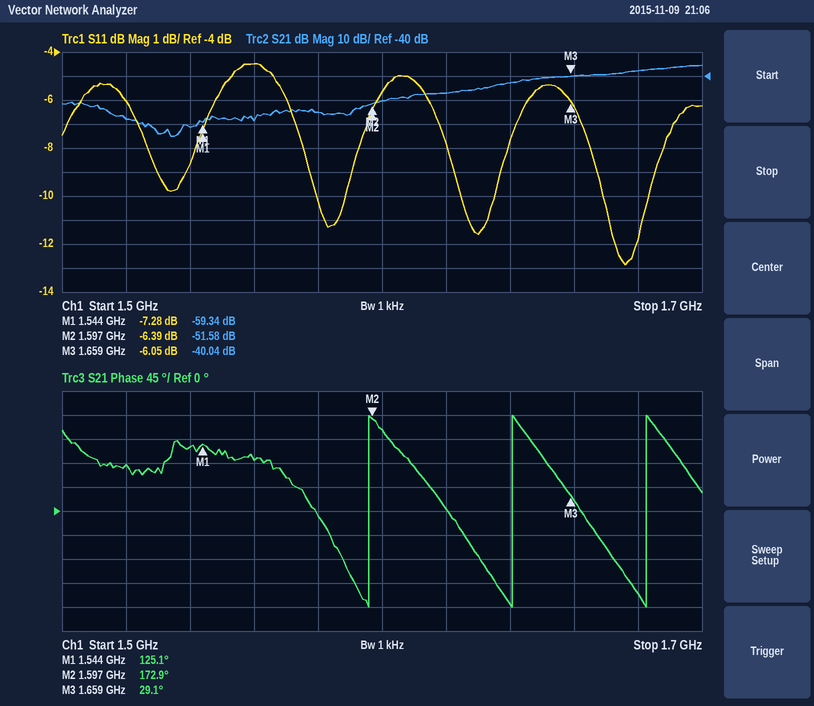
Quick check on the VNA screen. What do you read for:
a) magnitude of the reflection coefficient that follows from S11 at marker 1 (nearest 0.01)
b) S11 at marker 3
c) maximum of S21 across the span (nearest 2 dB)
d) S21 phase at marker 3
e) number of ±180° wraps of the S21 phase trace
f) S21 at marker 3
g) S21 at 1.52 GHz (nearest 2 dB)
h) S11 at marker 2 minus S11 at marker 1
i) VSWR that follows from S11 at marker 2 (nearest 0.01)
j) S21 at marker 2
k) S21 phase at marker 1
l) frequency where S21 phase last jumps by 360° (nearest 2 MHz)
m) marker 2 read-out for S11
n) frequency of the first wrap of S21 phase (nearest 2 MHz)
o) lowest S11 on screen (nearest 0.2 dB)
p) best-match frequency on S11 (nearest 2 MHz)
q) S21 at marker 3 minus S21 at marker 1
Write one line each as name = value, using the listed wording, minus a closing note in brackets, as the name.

magnitude of the reflection coefficient that follows from S11 at marker 1 = 0.43
S11 at marker 3 = -6.05 dB
maximum of S21 across the span = -36 dB
S21 phase at marker 3 = 29.1°
number of ±180° wraps of the S21 phase trace = 3
S21 at marker 3 = -40.04 dB
S21 at 1.52 GHz = -58 dB
S11 at marker 2 minus S11 at marker 1 = 0.89 dB
VSWR that follows from S11 at marker 2 = 2.84
S21 at marker 2 = -51.58 dB
S21 phase at marker 1 = 125.1°
frequency where S21 phase last jumps by 360° = 1.682 GHz
marker 2 read-out for S11 = -6.39 dB
frequency of the first wrap of S21 phase = 1.596 GHz
lowest S11 on screen = -12.8 dB
best-match frequency on S11 = 1.676 GHz
S21 at marker 3 minus S21 at marker 1 = 19.30 dB
